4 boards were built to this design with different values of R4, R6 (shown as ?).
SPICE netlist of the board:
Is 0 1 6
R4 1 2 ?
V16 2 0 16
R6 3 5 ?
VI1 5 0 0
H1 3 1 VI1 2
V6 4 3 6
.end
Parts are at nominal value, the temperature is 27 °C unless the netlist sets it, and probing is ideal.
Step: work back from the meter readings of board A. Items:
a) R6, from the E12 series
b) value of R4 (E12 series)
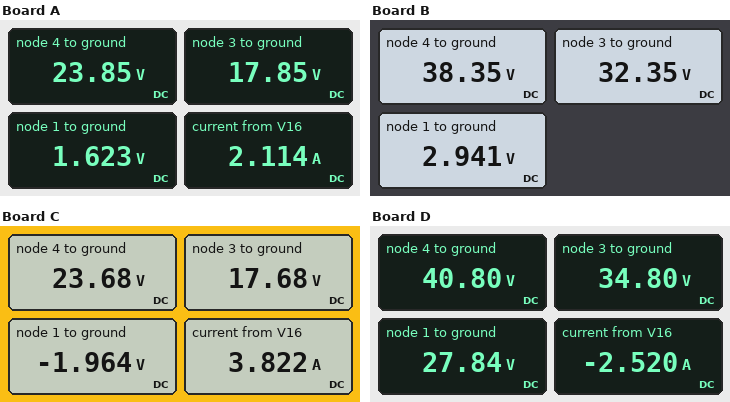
2.2 Ω
6.8 Ω
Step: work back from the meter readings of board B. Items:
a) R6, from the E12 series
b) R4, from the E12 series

2.2 Ω
1.5 Ω
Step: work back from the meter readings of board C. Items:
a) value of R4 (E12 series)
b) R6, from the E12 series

4.7 Ω
1.8 Ω
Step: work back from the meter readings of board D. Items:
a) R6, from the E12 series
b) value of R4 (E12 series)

10 Ω
4.7 Ω
